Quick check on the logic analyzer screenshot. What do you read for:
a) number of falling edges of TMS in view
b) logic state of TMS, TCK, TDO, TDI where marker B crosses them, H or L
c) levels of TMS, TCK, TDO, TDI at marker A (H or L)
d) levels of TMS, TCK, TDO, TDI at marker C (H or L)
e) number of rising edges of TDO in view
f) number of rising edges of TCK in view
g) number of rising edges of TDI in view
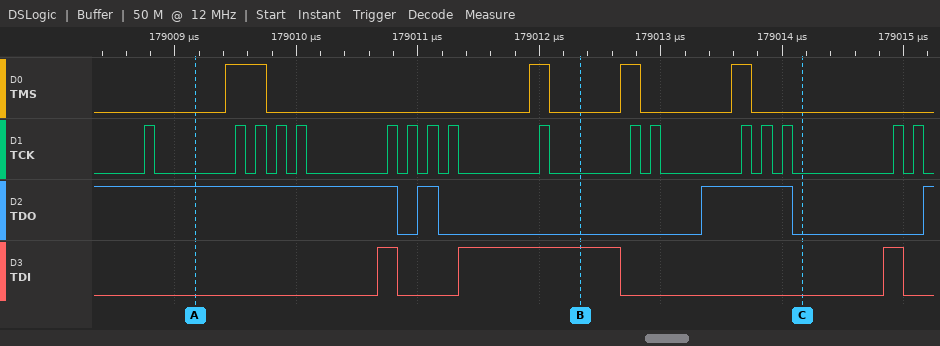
4
TMS=L, TCK=L, TDO=L, TDI=H
TMS=L, TCK=L, TDO=H, TDI=L
TMS=L, TCK=L, TDO=L, TDI=L
3
17
3
